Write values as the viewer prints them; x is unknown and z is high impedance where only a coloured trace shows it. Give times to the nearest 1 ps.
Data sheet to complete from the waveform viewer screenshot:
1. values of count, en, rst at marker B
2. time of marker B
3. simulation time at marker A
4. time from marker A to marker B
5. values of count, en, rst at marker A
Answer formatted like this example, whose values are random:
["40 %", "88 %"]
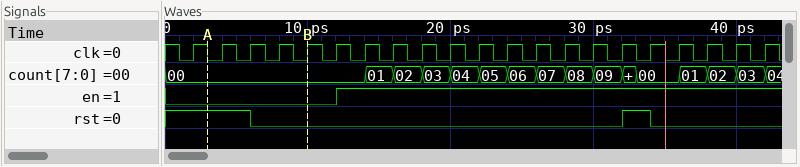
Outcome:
["count=00, en=0, rst=0", "10 ps", "3 ps", "7 ps", "count=00, en=0, rst=1"]
